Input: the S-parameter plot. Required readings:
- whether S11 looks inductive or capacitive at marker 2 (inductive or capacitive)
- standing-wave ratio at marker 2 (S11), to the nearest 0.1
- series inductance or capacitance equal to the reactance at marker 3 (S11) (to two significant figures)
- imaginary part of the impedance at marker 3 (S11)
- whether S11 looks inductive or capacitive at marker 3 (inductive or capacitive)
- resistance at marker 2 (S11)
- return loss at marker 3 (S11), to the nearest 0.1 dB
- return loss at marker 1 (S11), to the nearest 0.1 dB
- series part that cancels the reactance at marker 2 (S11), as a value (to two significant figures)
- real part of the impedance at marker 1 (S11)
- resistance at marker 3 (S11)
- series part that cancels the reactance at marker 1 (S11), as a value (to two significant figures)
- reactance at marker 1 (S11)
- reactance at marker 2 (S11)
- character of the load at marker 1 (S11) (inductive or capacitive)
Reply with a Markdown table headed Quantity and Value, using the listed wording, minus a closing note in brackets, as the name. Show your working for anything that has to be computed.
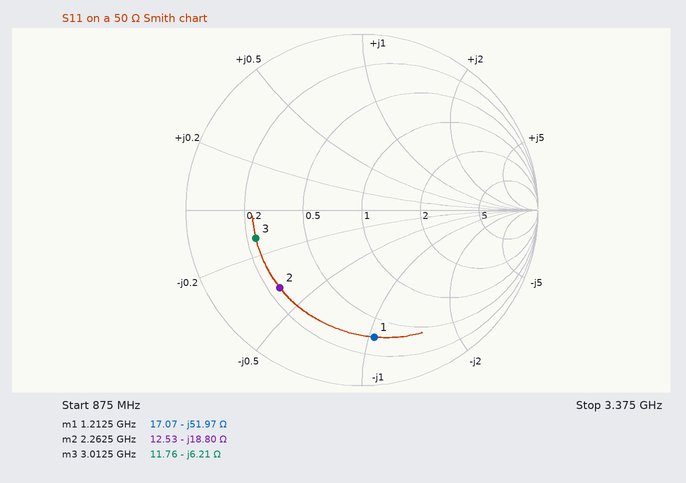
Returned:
| Quantity | Value |
|---|---|
| whether S11 looks inductive or capacitive at marker 2 | capacitive |
| standing-wave ratio at marker 2 (S11), to the nearest 0.1 | 4.6 |
| series inductance or capacitance equal to the reactance at marker 3 (S11) | C = 1/(2π × 3.0125 GHz × 6.21 Ω) ≈ 8.5 pF |
| imaginary part of the impedance at marker 3 | -6.21 Ω |
| whether S11 looks inductive or capacitive at marker 3 | capacitive |
| resistance at marker 2 | 12.53 Ω |
| return loss at marker 3 (S11), to the nearest 0.1 dB | 4.1 dB |
| return loss at marker 1 (S11), to the nearest 0.1 dB | 2.8 dB |
| series part that cancels the reactance at marker 2 (S11), as a value | L = 18.8 Ω/(2π × 2.2625 GHz) ≈ 1.3 nH |
| real part of the impedance at marker 1 | 17.07 Ω |
| resistance at marker 3 | 11.76 Ω |
| series part that cancels the reactance at marker 1 (S11), as a value | L = 51.97 Ω/(2π × 1.2125 GHz) ≈ 6.8 nH |
| reactance at marker 1 | -51.97 Ω |
| reactance at marker 2 | -18.80 Ω |
| character of the load at marker 1 (S11) | capacitive |
